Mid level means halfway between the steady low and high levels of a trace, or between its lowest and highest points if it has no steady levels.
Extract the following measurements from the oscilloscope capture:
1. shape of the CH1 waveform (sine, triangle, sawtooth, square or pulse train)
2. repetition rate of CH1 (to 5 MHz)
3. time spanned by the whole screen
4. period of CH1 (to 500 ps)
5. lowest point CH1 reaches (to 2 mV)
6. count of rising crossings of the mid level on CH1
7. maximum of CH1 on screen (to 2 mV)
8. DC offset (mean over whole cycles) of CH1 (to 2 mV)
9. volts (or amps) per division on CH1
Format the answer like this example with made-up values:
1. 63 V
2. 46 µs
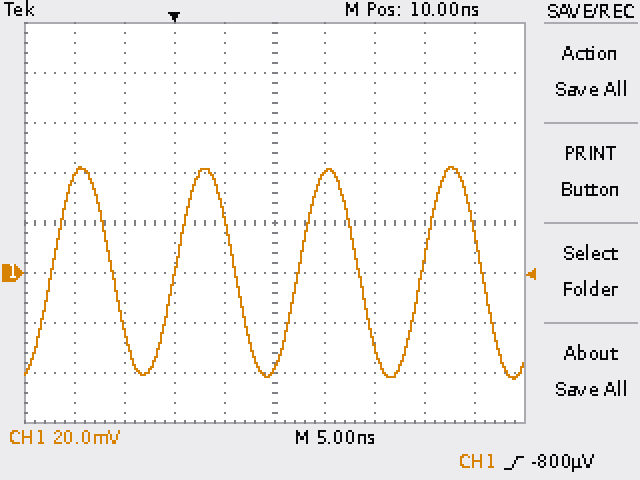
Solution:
1. sine
2. 80 MHz
3. 50 ns
4. 12.5 ns
5. -42 mV
6. 4
7. 42 mV
8. 0 mV
9. 20 mV
